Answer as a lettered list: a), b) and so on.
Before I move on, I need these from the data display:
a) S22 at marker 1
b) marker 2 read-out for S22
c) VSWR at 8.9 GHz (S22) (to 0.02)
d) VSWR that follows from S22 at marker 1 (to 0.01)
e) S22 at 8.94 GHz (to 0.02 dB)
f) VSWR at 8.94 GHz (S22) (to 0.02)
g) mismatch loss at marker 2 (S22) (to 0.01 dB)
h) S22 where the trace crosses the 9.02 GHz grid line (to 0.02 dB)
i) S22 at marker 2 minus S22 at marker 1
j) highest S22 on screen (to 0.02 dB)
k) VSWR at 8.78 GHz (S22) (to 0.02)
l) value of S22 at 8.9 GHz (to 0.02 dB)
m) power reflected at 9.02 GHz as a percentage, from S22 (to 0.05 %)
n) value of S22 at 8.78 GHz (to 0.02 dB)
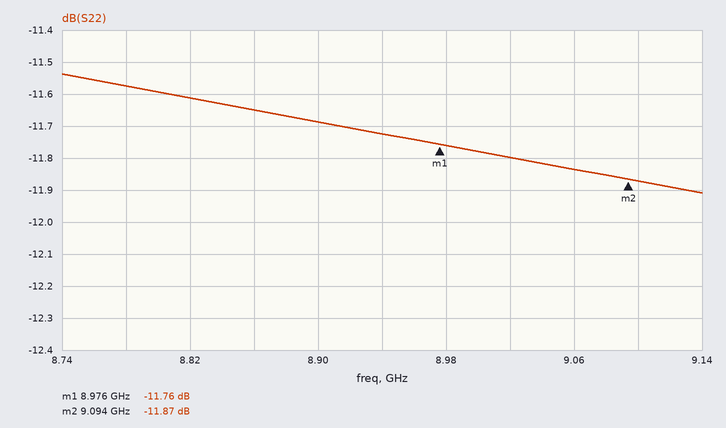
a) -11.76 dB
b) -11.87 dB
c) 1.70
d) 1.70
e) -11.72 dB
f) 1.70
g) 0.29 dB
h) -11.80 dB
i) -0.11 dB
j) -11.54 dB
k) 1.72
l) -11.68 dB
m) 6.60 %
n) -11.58 dB
